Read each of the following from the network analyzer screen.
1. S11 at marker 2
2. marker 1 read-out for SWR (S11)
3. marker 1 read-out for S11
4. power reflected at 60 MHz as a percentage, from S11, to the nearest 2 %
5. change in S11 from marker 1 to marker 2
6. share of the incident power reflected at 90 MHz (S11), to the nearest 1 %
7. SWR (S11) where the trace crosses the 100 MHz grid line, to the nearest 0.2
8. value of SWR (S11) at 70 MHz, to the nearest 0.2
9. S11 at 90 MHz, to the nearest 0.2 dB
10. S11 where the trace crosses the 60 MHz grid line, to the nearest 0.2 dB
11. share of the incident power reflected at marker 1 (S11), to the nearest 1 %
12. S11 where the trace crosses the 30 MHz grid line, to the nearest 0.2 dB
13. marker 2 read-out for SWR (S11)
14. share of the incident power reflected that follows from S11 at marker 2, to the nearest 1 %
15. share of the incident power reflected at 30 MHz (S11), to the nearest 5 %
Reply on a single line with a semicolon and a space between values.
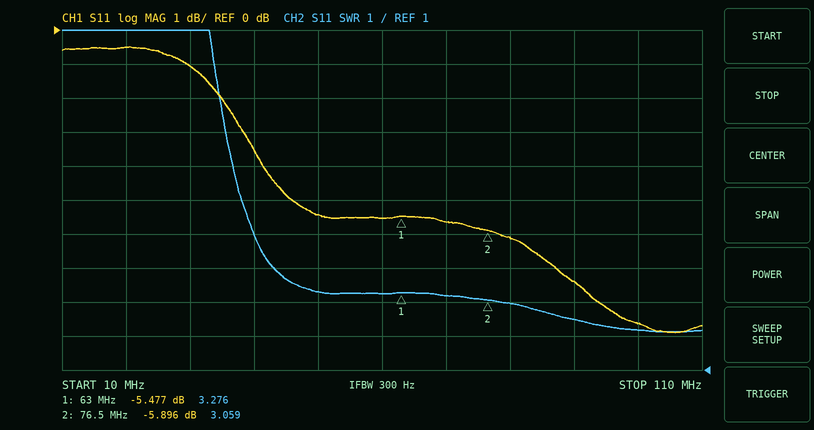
-5.896 dB; 3.276; -5.477 dB; 28 %; -0.419 dB; 18 %; 2.2; 3.2; -7.4 dB; -5.6 dB; 28 %; -1.0 dB; 3.059; 26 %; 80 %
